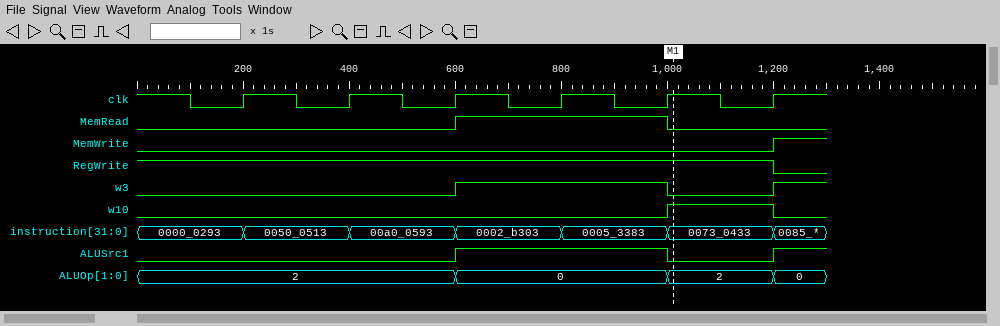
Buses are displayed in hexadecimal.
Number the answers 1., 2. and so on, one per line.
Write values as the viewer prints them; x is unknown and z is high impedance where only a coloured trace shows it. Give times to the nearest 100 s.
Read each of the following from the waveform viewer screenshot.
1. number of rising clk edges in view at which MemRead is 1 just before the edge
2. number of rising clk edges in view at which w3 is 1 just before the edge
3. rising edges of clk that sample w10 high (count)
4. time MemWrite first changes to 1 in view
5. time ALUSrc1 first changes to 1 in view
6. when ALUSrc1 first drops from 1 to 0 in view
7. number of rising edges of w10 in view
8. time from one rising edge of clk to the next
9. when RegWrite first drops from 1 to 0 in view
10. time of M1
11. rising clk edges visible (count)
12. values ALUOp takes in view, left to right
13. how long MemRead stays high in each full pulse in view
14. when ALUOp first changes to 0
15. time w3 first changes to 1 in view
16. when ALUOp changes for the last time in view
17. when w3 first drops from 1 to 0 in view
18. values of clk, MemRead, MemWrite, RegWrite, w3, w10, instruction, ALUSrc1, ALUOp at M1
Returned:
1. 2
2. 2
3. 1
4. 1200 s
5. 600 s
6. 1000 s
7. 1
8. 200 s
9. 1200 s
10. 1000 s
11. 6
12. 2, 0, 2, 0
13. 400 s
14. 600 s
15. 600 s
16. 1200 s
17. 1000 s
18. clk=1, MemRead=0, MemWrite=0, RegWrite=1, w3=0, w10=1, instruction=0073_0433, ALUSrc1=0, ALUOp=2
